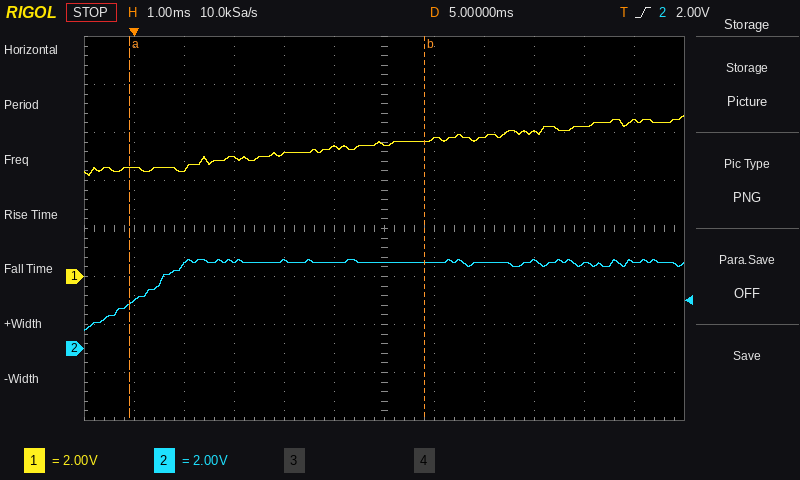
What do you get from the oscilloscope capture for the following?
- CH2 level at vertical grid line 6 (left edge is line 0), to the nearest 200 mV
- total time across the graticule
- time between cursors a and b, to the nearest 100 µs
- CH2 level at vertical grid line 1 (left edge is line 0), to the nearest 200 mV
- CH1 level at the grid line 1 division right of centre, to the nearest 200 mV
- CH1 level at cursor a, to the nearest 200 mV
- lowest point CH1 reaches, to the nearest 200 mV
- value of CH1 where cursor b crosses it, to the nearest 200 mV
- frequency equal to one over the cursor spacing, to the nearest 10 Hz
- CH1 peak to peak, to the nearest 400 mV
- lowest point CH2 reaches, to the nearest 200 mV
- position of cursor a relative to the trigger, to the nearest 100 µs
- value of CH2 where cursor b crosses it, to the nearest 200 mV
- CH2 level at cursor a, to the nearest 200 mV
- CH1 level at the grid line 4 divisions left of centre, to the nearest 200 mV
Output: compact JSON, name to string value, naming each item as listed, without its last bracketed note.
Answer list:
{"CH2 level at vertical grid line 6 (left edge is line 0), to the nearest 200 mV": "3.6 V", "total time across the graticule": "12 ms", "time between cursors a and b, to the nearest 100 µs": "5.9 ms", "CH2 level at vertical grid line 1 (left edge is line 0), to the nearest 200 mV": "2.0 V", "CH1 level at the grid line 1 division right of centre, to the nearest 200 mV": "5.8 V", "CH1 level at cursor a, to the nearest 200 mV": "4.6 V", "lowest point CH1 reaches, to the nearest 200 mV": "4.2 V", "value of CH1 where cursor b crosses it, to the nearest 200 mV": "5.6 V", "frequency equal to one over the cursor spacing, to the nearest 10 Hz": "170 Hz", "CH1 peak to peak, to the nearest 400 mV": "2.4 V", "lowest point CH2 reaches, to the nearest 200 mV": "800 mV", "position of cursor a relative to the trigger, to the nearest 100 µs": "-100 µs", "value of CH2 where cursor b crosses it, to the nearest 200 mV": "3.6 V", "CH2 level at cursor a, to the nearest 200 mV": "1.8 V", "CH1 level at the grid line 4 divisions left of centre, to the nearest 200 mV": "4.4 V"}
